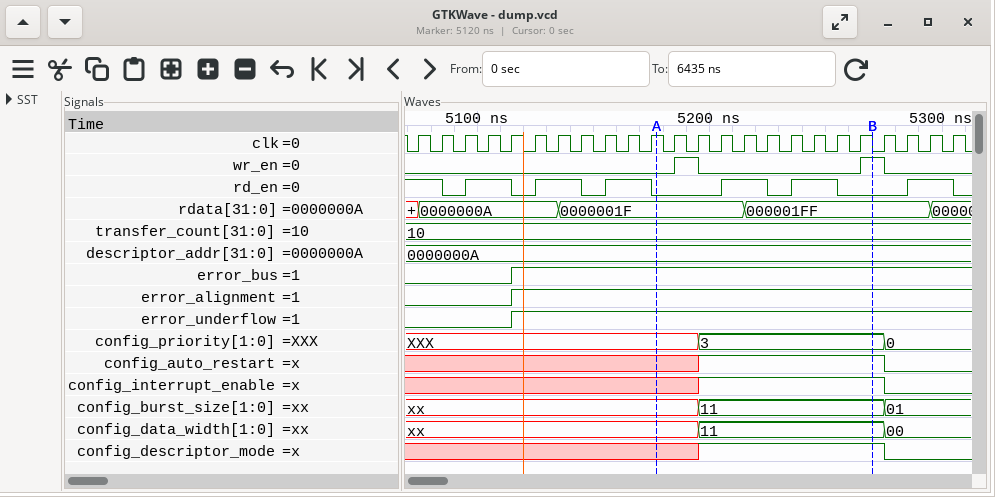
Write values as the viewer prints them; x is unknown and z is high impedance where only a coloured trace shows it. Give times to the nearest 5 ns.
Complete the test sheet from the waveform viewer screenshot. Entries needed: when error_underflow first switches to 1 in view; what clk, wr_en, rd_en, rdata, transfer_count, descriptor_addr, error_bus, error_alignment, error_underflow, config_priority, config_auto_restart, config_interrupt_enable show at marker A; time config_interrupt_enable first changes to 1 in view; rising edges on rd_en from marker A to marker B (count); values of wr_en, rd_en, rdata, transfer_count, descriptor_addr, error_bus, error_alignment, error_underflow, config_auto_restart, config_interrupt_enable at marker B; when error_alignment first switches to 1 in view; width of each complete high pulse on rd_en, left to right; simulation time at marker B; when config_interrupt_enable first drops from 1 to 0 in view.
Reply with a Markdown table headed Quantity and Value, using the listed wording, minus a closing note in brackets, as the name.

| Quantity | Value |
|---|---|
| when error_underflow first switches to 1 in view | 5115 ns |
| what clk, wr_en, rd_en, rdata, transfer_count, descriptor_addr, error_bus, error_alignment, error_underflow, config_priority, config_auto_restart, config_interrupt_enable show at marker A | clk=1, wr_en=0, rd_en=0, rdata=0000001F, transfer_count=10, descriptor_addr=0000000A, error_bus=1, error_alignment=1, error_underflow=1, config_priority=XXX, config_auto_restart=x, config_interrupt_enable=x |
| time config_interrupt_enable first changes to 1 in view | 5195 ns |
| rising edges on rd_en from marker A to marker B | 2 |
| values of wr_en, rd_en, rdata, transfer_count, descriptor_addr, error_bus, error_alignment, error_underflow, config_auto_restart, config_interrupt_enable at marker B | wr_en=1, rd_en=0, rdata=000001FF, transfer_count=10, descriptor_addr=0000000A, error_bus=1, error_alignment=1, error_underflow=1, config_auto_restart=1, config_interrupt_enable=1 |
| when error_alignment first switches to 1 in view | 5115 ns |
| width of each complete high pulse on rd_en, left to right | 20 ns, 20 ns, 20 ns, 20 ns, 20 ns, 20 ns |
| simulation time at marker B | 5270 ns |
| when config_interrupt_enable first drops from 1 to 0 in view | 5275 ns |
